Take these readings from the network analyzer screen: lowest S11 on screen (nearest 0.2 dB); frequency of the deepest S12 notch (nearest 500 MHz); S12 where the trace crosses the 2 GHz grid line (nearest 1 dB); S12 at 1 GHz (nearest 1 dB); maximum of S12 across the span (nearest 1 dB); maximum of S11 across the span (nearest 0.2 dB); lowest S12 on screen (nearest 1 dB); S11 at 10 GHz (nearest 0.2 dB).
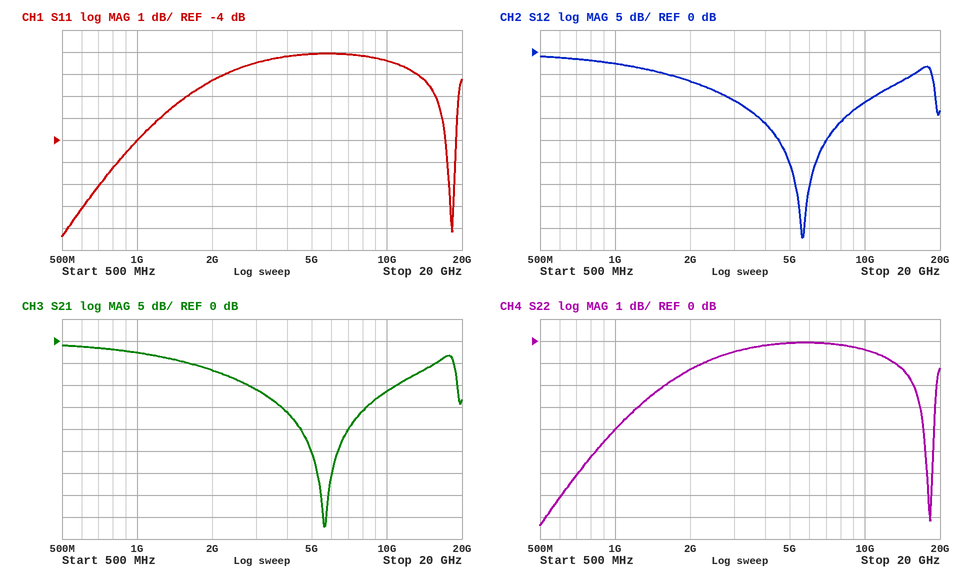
-8.4 dB
5.5 GHz
-7 dB
-3 dB
-1 dB
0.0 dB
-42 dB
-0.4 dB
